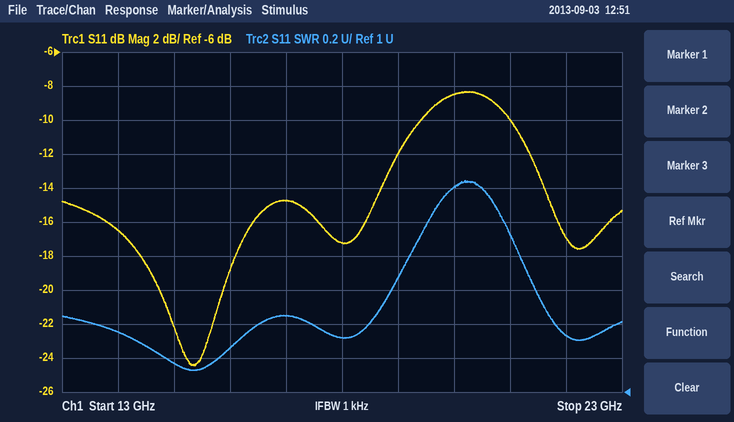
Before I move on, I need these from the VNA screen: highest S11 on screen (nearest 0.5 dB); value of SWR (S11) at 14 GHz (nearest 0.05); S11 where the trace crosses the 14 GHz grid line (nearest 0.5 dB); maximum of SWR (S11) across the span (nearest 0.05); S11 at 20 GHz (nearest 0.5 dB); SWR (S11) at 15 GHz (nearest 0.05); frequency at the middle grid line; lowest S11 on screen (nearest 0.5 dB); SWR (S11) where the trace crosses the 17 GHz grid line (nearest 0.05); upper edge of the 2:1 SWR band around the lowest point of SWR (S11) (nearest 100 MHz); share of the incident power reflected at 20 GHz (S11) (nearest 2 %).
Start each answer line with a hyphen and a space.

- -8.5 dB
- 1.35
- -16.5 dB
- 2.25
- -8.5 dB
- 1.15
- 18 GHz
- -24.5 dB
- 1.45
- 19.5 GHz
- 14 %
